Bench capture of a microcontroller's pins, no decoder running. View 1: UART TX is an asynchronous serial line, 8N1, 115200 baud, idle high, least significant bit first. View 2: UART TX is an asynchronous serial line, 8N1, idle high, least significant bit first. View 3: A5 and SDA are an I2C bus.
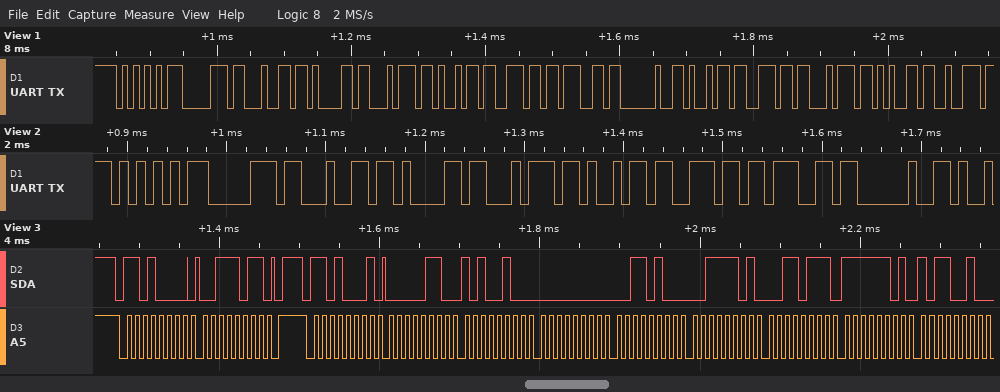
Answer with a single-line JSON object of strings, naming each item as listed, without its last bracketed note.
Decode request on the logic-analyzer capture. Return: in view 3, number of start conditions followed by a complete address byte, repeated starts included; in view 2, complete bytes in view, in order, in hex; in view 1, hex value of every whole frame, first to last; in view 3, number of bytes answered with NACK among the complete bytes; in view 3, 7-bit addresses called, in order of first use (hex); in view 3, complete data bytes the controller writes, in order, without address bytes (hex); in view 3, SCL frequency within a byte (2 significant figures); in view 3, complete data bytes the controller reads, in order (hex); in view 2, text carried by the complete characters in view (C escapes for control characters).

{"in view 3, number of start conditions followed by a complete address byte, repeated starts included": "2", "in view 2, complete bytes in view, in order, in hex": "0x55 0x70 0x64 0x61 0x74 0x69 0x6E 0x67 0x20", "in view 1, hex value of every whole frame, first to last": "0x55 0x70 0x64 0x61 0x74 0x69 0x6E 0x67 0x20 0x69 0x6E 0x74 0x65 0x72", "in view 3, number of bytes answered with NACK among the complete bytes": "0", "in view 3, 7-bit addresses called, in order of first use": "0x68", "in view 3, complete data bytes the controller writes, in order, without address bytes": "3B", "in view 3, SCL frequency within a byte": "100 kHz", "in view 3, complete data bytes the controller reads, in order": "06 A4 00 34 3D 37 FD B2", "in view 2, text carried by the complete characters in view": "\"Updating \""}
